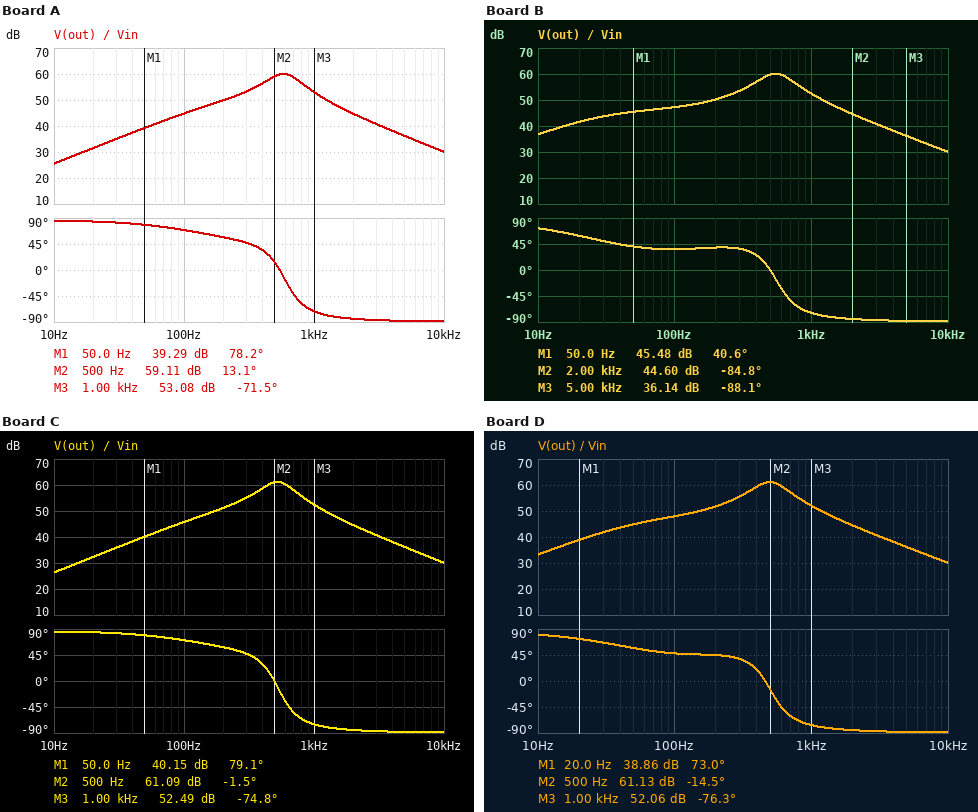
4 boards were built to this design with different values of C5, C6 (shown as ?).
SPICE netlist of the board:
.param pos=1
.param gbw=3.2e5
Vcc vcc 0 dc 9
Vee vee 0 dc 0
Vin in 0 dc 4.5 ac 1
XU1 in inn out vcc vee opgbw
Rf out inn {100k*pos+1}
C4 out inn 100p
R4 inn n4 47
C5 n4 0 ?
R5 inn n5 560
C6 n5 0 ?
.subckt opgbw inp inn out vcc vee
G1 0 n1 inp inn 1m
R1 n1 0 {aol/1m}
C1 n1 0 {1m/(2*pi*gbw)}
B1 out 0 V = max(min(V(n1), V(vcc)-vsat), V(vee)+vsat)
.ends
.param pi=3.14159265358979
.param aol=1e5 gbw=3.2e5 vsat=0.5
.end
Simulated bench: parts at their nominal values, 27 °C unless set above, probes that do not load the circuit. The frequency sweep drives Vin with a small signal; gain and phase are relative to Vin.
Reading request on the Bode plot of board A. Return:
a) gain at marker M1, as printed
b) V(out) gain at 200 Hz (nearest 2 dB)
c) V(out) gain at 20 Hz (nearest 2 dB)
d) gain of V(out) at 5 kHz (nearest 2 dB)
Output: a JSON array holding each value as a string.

["39.29 dB", "50 dB", "32 dB", "36 dB"]
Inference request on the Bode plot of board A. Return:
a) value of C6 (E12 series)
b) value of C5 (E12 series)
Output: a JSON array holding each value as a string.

["1.8 µF", "1.2 µF"]
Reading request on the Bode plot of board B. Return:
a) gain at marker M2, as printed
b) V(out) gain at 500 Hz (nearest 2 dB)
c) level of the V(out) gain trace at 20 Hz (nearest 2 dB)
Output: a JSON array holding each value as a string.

["44.60 dB", "60 dB", "42 dB"]
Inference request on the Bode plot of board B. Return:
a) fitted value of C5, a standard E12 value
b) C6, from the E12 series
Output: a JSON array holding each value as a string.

["1.5 µF", "10 µF"]
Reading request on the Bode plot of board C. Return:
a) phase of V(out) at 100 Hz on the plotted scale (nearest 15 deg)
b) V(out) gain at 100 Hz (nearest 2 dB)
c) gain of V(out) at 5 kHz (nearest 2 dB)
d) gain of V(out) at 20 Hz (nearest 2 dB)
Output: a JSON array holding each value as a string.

["75 deg", "46 dB", "36 dB", "32 dB"]
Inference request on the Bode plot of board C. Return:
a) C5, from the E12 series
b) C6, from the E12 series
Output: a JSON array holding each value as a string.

["1.5 µF", "1.8 µF"]
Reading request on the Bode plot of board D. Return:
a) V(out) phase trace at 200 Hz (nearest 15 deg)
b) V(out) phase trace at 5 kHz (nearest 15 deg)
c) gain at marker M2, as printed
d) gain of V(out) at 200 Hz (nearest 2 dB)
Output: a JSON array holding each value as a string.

["45 deg", "-90 deg", "61.13 dB", "52 dB"]
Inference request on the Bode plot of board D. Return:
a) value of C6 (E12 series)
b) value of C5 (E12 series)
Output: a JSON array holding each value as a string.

["5.6 µF", "1.8 µF"]
